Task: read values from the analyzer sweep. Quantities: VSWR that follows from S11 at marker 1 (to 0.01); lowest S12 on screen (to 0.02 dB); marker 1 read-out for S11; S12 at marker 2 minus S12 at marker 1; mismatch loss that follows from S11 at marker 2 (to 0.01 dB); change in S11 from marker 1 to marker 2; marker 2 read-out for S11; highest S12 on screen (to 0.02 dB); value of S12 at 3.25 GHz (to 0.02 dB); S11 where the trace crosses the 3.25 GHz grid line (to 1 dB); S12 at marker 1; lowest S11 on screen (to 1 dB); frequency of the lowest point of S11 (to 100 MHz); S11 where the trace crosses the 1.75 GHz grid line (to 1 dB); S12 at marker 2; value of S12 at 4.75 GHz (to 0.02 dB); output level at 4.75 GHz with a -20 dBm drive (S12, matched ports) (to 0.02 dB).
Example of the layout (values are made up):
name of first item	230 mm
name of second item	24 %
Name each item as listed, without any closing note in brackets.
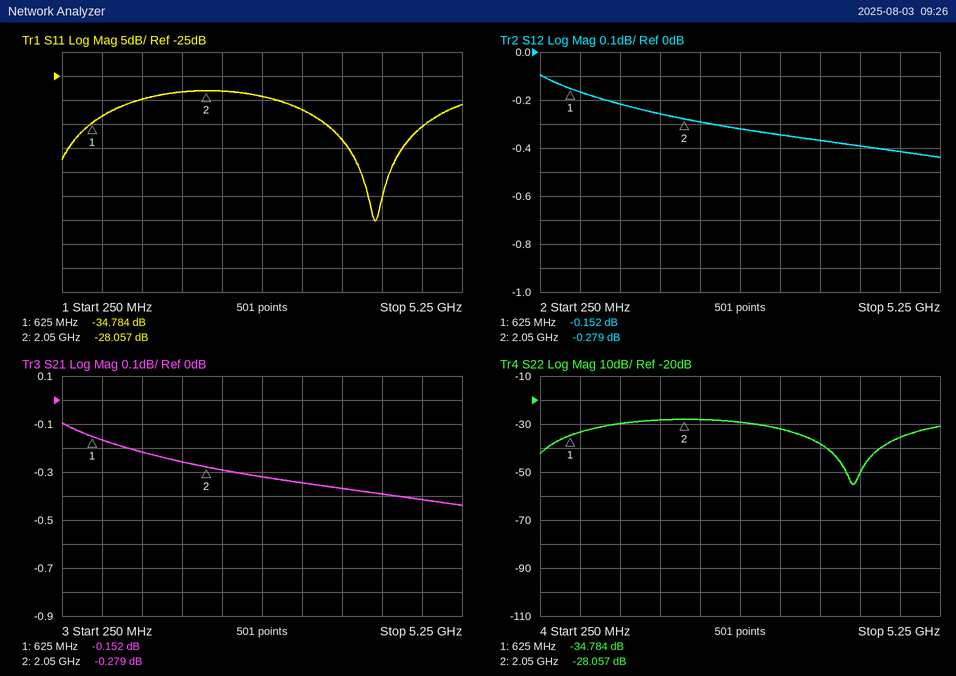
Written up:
VSWR that follows from S11 at marker 1	1.04
lowest S12 on screen	-0.44 dB
marker 1 read-out for S11	-34.784 dB
S12 at marker 2 minus S12 at marker 1	-0.127 dB
mismatch loss that follows from S11 at marker 2	0.01 dB
change in S11 from marker 1 to marker 2	6.727 dB
marker 2 read-out for S11	-28.057 dB
highest S12 on screen	-0.10 dB
value of S12 at 3.25 GHz	-0.34 dB
S11 where the trace crosses the 3.25 GHz grid line	-32 dB
S12 at marker 1	-0.152 dB
lowest S11 on screen	-55 dB
frequency of the lowest point of S11	4.2 GHz
S11 where the trace crosses the 1.75 GHz grid line	-28 dB
S12 at marker 2	-0.279 dB
value of S12 at 4.75 GHz	-0.42 dB
output level at 4.75 GHz with a -20 dBm drive (S12, matched ports)	-20.42 dBm
